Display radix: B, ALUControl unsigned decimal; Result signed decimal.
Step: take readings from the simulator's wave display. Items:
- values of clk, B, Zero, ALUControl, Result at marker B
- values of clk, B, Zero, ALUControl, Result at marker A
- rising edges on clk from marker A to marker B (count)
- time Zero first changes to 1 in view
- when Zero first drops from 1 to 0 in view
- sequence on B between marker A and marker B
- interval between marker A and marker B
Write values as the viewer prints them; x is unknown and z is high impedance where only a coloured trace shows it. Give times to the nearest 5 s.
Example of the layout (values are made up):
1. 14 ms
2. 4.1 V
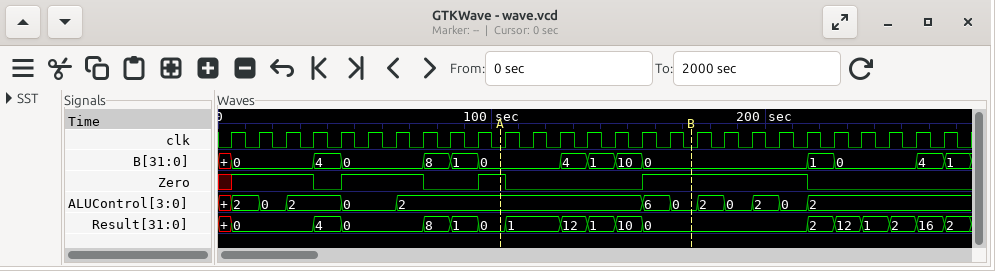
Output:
1. clk=0, B=0, Zero=1, ALUControl=0, Result=0
2. clk=0, B=0, Zero=1, ALUControl=2, Result=0
3. 7
4. 5 s
5. 35 s
6. 0, 4, 1, 10, 0
7. 70 s
